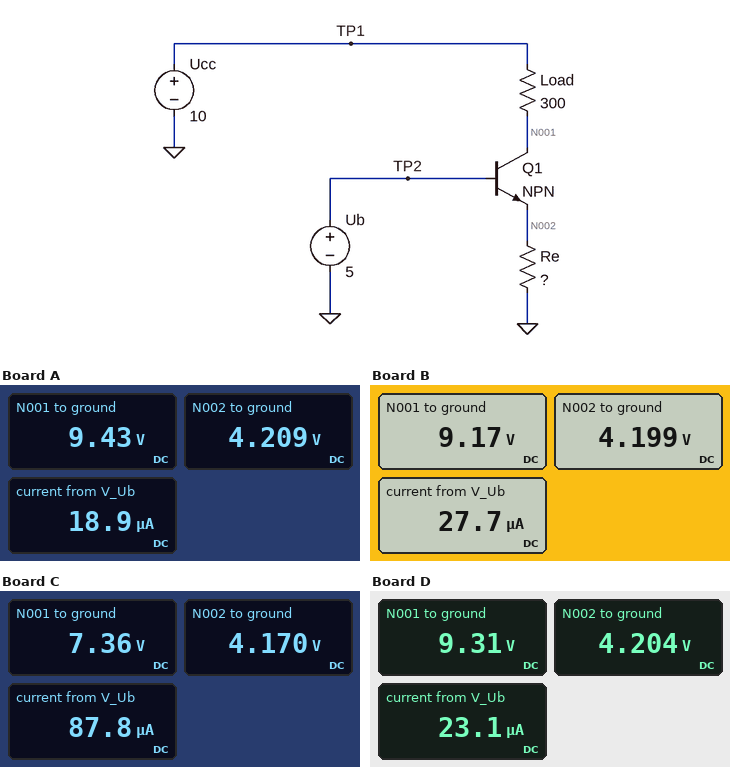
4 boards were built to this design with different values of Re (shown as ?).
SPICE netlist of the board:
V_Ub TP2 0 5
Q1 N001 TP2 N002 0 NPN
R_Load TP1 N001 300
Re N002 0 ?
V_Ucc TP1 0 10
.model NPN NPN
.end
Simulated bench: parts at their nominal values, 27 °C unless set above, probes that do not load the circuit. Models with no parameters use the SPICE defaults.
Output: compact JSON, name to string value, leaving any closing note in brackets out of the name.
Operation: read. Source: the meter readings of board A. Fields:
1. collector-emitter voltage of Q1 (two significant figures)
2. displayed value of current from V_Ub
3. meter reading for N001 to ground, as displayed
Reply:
{"collector-emitter voltage of Q1": "5.2 V", "displayed value of current from V_Ub": "18.9 µA", "meter reading for N001 to ground, as displayed": "9.43 V"}
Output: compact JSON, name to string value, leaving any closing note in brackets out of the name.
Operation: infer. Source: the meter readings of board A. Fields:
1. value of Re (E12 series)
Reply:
{"value of Re": "2.2 kΩ"}
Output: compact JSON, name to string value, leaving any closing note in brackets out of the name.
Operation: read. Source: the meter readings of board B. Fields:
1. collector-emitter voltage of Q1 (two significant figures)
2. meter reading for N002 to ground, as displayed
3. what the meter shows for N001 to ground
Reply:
{"collector-emitter voltage of Q1": "5.0 V", "meter reading for N002 to ground, as displayed": "4.199 V", "what the meter shows for N001 to ground": "9.17 V"}
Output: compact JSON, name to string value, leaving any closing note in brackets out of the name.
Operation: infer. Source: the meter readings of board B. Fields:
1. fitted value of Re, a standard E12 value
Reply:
{"fitted value of Re, a standard E12 value": "1.5 kΩ"}
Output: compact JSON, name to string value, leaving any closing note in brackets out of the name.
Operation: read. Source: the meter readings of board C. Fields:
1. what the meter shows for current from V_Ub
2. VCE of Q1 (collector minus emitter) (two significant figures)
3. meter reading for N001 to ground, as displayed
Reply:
{"what the meter shows for current from V_Ub": "87.8 µA", "VCE of Q1 (collector minus emitter)": "3.2 V", "meter reading for N001 to ground, as displayed": "7.36 V"}
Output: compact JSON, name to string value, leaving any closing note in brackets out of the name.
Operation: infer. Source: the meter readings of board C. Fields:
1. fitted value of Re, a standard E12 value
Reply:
{"fitted value of Re, a standard E12 value": "470 Ω"}
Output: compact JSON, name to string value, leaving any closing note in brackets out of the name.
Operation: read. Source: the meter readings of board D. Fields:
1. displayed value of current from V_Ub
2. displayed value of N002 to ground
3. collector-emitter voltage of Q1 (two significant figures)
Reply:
{"displayed value of current from V_Ub": "23.1 µA", "displayed value of N002 to ground": "4.204 V", "collector-emitter voltage of Q1": "5.1 V"}
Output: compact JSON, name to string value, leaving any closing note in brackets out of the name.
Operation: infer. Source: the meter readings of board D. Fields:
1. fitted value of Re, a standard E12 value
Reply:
{"fitted value of Re, a standard E12 value": "1.8 kΩ"}
